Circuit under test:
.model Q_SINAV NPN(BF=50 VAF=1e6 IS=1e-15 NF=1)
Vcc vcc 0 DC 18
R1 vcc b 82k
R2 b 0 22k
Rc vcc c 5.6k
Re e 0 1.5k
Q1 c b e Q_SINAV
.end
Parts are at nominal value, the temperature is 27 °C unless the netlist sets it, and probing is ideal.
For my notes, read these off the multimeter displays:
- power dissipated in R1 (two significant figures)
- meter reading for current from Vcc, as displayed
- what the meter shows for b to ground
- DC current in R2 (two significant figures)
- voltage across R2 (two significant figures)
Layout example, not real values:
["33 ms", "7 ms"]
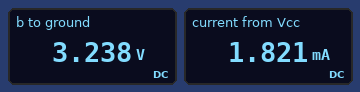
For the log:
["2.7 mW", "1.821 mA", "3.238 V", "150 µA", "3.2 V"]
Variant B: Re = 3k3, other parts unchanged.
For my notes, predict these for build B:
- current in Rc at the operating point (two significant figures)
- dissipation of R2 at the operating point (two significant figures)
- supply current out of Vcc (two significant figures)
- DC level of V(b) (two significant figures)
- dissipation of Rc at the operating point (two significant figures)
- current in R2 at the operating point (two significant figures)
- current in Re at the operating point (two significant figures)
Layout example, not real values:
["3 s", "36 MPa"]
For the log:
["830 µA", "560 µW", "1.0 mA", "3.5 V", "3.9 mW", "160 µA", "850 µA"]
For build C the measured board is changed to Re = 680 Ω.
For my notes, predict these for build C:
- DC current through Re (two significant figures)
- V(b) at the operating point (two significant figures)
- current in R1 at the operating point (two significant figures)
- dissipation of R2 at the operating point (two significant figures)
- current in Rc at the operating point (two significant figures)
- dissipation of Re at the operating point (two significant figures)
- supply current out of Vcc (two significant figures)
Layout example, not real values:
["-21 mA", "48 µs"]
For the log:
["2.9 mA", "2.7 V", "190 µA", "330 µW", "2.8 mA", "5.7 mW", "3.0 mA"]
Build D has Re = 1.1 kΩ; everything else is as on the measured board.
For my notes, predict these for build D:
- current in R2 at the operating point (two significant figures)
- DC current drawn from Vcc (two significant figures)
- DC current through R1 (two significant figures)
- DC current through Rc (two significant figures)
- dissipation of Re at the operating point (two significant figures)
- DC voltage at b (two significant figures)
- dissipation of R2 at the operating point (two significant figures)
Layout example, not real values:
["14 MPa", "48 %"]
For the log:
["140 µA", "2.3 mA", "180 µA", "2.1 mA", "5.0 mW", "3.1 V", "430 µW"]
